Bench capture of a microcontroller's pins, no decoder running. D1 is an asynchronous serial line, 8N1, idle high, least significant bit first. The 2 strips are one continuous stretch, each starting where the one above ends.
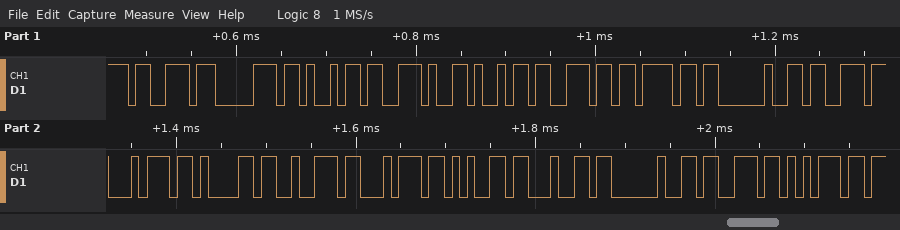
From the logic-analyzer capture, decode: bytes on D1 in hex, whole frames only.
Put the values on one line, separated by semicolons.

0x73 0x70 0x69 0x2E 0x69 0x6E 0x6F 0x20 0x73 0x74 0x61 0x72 0x74 0x65 0x64 0x20 0x73 0x75
